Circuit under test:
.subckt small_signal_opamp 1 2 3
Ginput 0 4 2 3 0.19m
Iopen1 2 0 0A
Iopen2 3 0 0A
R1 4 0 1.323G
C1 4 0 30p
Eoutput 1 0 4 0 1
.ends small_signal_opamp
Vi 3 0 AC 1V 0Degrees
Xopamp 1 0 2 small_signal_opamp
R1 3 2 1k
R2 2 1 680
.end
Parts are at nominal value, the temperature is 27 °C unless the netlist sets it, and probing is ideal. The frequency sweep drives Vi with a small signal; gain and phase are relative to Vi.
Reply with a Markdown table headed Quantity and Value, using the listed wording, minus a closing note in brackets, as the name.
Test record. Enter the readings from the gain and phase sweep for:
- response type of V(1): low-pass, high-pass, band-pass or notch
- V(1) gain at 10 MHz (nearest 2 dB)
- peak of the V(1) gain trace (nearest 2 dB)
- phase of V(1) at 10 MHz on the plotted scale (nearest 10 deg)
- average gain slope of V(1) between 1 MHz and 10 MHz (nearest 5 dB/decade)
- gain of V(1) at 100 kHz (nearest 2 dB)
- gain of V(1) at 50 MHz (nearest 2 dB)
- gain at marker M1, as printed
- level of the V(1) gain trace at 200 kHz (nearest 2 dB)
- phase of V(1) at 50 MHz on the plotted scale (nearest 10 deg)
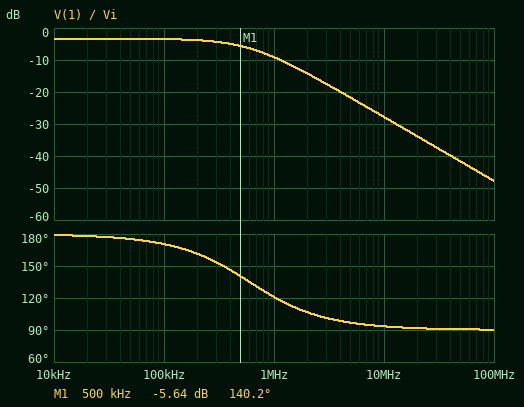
| Quantity | Value |
|---|---|
| response type of V(1): low-pass, high-pass, band-pass or notch | low-pass |
| V(1) gain at 10 MHz | -28 dB |
| peak of the V(1) gain trace | -4 dB |
| phase of V(1) at 10 MHz on the plotted scale | 90 deg |
| average gain slope of V(1) between 1 MHz and 10 MHz | -20 dB/decade |
| gain of V(1) at 100 kHz | -4 dB |
| gain of V(1) at 50 MHz | -42 dB |
| gain at marker M1, as printed | -5.64 dB |
| level of the V(1) gain trace at 200 kHz | -4 dB |
| phase of V(1) at 50 MHz on the plotted scale | 90 deg |
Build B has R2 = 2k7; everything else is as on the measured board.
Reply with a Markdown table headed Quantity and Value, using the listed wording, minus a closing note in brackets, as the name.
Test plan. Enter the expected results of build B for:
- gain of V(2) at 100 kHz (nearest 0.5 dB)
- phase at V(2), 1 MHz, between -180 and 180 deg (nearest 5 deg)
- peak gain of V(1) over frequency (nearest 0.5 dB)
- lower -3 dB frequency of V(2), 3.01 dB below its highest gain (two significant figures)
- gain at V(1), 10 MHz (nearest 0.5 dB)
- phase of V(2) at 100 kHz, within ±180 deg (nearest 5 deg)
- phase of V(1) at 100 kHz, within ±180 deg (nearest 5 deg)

| Quantity | Value |
|---|---|
| gain of V(2) at 100 kHz | -12.0 dB |
| phase at V(2), 1 MHz, between -180 and 180 deg | 15 deg |
| peak gain of V(1) over frequency | 8.5 dB |
| lower -3 dB frequency of V(2), 3.01 dB below its highest gain | 270 kHz |
| gain at V(1), 10 MHz | -22.5 dB |
| phase of V(2) at 100 kHz, within ±180 deg | 70 deg |
| phase of V(1) at 100 kHz, within ±180 deg | 160 deg |
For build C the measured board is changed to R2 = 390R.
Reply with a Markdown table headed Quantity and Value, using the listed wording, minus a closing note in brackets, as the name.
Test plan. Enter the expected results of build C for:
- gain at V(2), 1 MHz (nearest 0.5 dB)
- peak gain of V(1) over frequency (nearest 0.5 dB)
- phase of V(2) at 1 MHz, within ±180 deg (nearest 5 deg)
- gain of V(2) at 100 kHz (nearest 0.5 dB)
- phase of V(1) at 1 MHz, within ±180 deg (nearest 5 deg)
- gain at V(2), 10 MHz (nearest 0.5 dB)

| Quantity | Value |
|---|---|
| gain at V(2), 1 MHz | -13.0 dB |
| peak gain of V(1) over frequency | -8.0 dB |
| phase of V(2) at 1 MHz, within ±180 deg | 35 deg |
| gain of V(2) at 100 kHz | -28.5 dB |
| phase of V(1) at 1 MHz, within ±180 deg | 125 deg |
| gain at V(2), 10 MHz | -11.0 dB |
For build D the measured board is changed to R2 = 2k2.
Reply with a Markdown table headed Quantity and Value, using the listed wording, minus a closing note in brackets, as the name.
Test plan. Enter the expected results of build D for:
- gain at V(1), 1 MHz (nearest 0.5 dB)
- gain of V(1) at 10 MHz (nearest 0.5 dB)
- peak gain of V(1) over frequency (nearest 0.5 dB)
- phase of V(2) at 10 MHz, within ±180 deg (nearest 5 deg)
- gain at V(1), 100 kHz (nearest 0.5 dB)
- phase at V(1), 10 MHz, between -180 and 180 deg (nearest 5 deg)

| Quantity | Value |
|---|---|
| gain at V(1), 1 MHz | -3.5 dB |
| gain of V(1) at 10 MHz | -23.0 dB |
| peak gain of V(1) over frequency | 7.0 dB |
| phase of V(2) at 10 MHz, within ±180 deg | 0 deg |
| gain at V(1), 100 kHz | 6.5 dB |
| phase at V(1), 10 MHz, between -180 and 180 deg | 90 deg |
